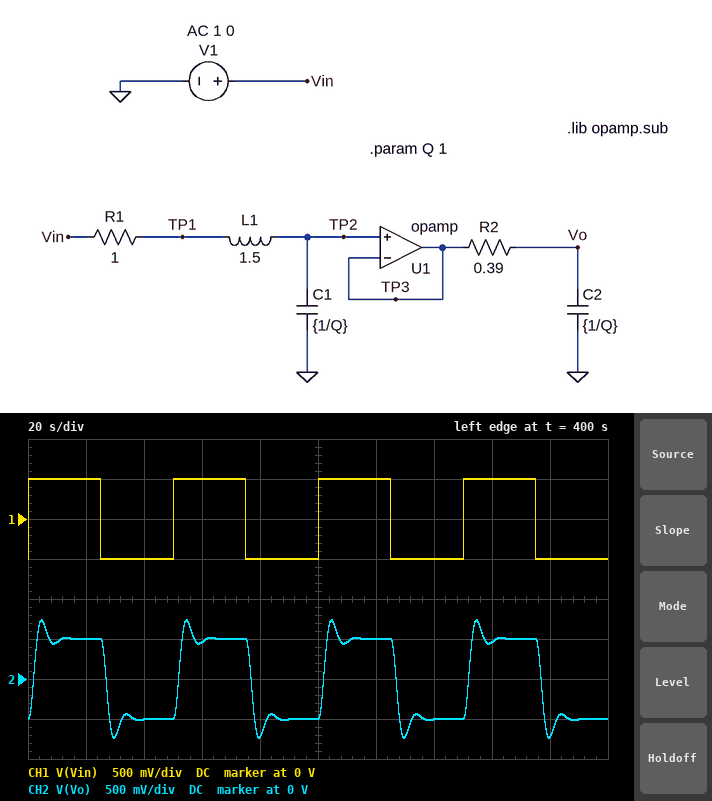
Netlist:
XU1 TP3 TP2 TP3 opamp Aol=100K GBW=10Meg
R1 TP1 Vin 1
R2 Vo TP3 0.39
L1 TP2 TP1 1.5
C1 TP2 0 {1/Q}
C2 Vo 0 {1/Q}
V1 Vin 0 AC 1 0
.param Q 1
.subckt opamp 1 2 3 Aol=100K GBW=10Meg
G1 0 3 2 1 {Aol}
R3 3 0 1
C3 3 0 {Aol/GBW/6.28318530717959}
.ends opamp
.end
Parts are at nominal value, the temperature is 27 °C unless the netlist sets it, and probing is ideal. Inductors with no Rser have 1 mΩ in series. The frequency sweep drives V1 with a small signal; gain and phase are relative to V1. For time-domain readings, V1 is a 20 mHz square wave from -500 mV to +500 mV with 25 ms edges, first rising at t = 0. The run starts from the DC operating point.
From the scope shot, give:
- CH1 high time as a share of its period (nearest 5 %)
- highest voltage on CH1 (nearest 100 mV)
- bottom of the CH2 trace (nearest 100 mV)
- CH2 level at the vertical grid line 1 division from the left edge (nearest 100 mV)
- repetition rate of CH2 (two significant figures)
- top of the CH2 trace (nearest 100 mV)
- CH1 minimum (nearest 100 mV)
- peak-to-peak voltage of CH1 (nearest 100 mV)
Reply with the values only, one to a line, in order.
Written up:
50 %
500 mV
-700 mV
500 mV
20 mHz
700 mV
-500 mV
1.0 V
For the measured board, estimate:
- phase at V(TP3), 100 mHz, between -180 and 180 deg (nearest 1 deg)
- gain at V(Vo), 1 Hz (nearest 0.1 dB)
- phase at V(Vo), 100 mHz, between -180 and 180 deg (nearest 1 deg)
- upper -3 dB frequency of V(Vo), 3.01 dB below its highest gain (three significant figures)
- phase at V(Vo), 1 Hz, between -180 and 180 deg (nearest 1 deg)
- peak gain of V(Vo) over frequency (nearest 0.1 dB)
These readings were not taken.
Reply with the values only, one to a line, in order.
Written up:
-57 deg
-43.8 dB
-71 deg
152 mHz
118 deg
2.3 dB
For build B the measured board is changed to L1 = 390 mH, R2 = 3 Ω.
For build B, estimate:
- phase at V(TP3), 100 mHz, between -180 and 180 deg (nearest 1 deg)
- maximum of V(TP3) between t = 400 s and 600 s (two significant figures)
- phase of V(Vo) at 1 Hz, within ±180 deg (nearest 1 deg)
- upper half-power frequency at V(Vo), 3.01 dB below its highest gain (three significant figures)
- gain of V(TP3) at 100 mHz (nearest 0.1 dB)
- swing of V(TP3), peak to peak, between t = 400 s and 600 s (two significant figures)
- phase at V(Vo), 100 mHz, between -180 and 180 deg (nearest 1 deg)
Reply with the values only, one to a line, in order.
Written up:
-37 deg
520 mV
117 deg
51.7 mHz
-0.5 dB
1.0 V
-99 deg
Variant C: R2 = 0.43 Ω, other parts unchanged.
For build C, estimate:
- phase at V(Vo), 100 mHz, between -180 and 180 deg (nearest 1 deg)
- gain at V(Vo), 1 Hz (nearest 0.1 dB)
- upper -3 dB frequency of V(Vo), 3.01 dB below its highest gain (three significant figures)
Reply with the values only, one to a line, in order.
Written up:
-72 deg
-44.5 dB
151 mHz
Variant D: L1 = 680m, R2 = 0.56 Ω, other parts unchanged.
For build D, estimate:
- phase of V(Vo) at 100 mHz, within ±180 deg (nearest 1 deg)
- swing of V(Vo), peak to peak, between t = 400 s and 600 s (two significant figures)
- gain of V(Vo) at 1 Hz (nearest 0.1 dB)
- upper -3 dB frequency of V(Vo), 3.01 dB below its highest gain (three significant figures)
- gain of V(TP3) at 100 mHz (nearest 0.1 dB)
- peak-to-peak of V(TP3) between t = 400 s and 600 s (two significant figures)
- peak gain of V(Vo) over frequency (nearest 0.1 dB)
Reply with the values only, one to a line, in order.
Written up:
-60 deg
1.1 V
-39.8 dB
187 mHz
0.3 dB
1.2 V
0 dB
